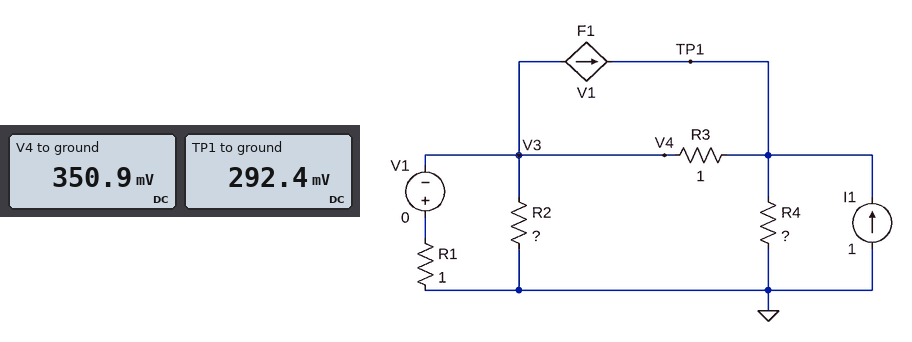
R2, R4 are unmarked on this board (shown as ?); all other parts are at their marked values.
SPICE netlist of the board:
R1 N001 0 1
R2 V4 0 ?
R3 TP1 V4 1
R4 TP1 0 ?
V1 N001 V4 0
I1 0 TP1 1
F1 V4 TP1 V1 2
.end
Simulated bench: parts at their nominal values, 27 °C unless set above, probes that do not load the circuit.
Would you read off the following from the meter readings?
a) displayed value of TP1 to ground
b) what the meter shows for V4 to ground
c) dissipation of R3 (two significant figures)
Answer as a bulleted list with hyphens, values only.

- 292.4 mV
- 350.9 mV
- 3.4 mW
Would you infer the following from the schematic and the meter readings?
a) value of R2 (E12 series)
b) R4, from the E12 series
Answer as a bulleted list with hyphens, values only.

- 1.2 Ω
- 0.82 Ω
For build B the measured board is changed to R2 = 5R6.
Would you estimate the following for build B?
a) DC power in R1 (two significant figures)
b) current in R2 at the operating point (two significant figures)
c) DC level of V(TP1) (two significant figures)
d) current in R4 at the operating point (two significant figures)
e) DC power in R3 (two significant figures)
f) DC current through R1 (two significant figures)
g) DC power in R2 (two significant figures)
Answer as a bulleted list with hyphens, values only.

- 510 mW
- 130 mA
- 130 mV
- 160 mA
- 350 mW
- 720 mA
- 92 mW
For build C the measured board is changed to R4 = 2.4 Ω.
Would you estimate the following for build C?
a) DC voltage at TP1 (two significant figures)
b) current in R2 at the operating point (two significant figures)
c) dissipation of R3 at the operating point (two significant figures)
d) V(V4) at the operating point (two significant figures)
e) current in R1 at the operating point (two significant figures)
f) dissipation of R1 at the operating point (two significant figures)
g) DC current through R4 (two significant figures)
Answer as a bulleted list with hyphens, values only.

- 380 mV
- 380 mA
- 5.8 mW
- 460 mV
- 460 mA
- 210 mW
- 160 mA
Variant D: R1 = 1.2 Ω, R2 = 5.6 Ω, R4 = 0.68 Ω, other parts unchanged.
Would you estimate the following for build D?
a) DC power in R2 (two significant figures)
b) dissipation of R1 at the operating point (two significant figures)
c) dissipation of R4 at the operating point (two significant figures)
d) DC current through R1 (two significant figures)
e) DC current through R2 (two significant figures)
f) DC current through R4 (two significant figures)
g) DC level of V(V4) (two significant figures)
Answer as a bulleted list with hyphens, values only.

- 77 mW
- 360 mW
- 76 mW
- 550 mA
- 120 mA
- 330 mA
- 660 mV
